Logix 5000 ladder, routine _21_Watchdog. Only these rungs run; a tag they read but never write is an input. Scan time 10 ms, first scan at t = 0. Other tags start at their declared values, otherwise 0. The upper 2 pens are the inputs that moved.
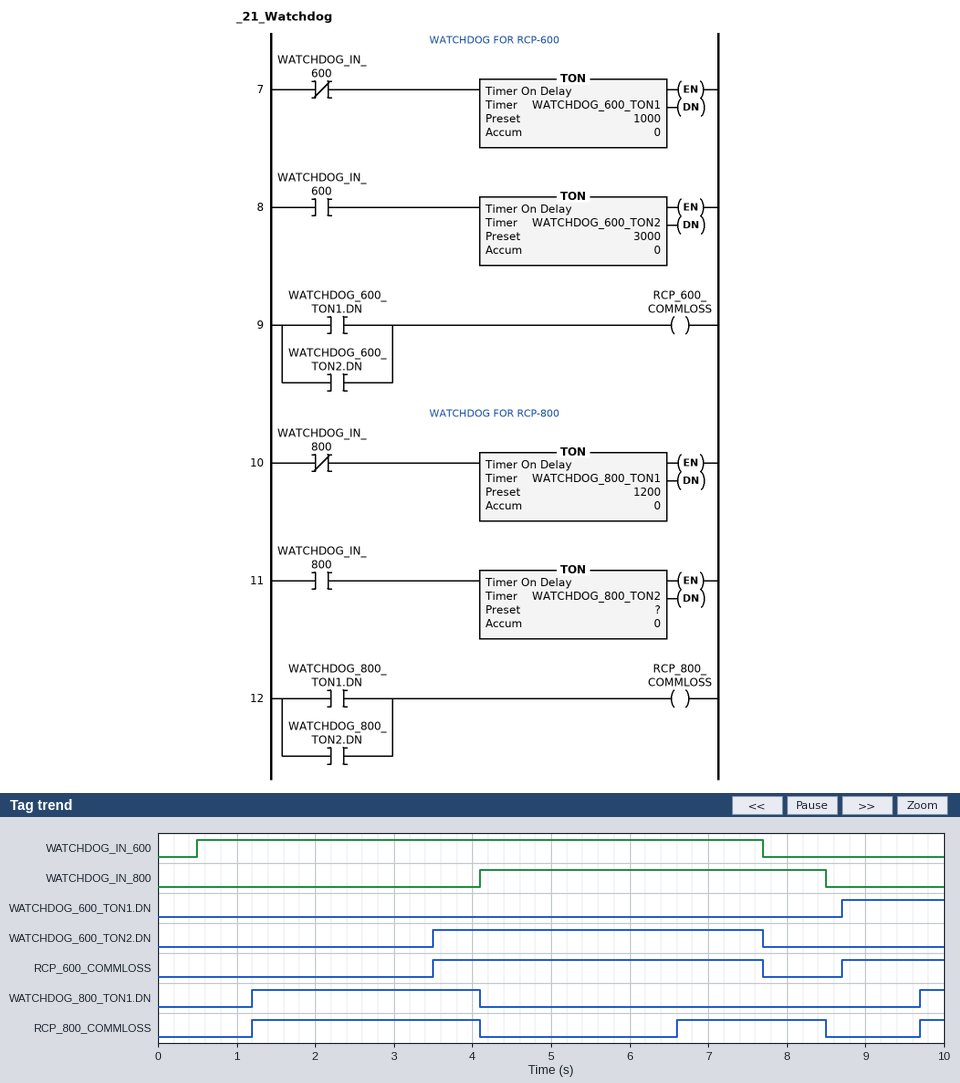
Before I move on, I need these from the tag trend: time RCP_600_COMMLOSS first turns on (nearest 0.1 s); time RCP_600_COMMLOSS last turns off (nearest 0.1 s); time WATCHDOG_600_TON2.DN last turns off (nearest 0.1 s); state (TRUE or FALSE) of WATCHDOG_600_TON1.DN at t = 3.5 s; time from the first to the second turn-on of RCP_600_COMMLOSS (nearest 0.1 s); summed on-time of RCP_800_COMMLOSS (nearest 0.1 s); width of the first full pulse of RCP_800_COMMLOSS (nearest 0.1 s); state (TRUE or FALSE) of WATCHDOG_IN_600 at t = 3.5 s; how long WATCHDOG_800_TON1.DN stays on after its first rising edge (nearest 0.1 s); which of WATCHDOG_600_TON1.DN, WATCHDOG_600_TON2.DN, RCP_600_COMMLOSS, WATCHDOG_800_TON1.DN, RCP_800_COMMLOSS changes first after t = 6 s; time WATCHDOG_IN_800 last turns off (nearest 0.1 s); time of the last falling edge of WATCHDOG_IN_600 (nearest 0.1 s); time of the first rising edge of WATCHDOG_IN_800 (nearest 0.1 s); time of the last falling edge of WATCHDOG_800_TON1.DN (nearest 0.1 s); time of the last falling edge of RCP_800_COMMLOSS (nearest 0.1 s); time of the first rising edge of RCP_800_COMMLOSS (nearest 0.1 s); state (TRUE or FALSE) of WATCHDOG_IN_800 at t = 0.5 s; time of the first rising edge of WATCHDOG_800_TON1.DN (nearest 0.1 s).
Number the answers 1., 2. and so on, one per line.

1. 3.5 s
2. 7.7 s
3. 7.7 s
4. FALSE
5. 5.2 s
6. 5.1 s
7. 2.9 s
8. TRUE
9. 2.9 s
10. RCP_800_COMMLOSS
11. 8.5 s
12. 7.7 s
13. 4.1 s
14. 4.1 s
15. 8.5 s
16. 1.2 s
17. FALSE
18. 1.2 s
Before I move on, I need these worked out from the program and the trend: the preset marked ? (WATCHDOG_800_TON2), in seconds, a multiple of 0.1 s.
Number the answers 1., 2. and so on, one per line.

1. 2.5 s
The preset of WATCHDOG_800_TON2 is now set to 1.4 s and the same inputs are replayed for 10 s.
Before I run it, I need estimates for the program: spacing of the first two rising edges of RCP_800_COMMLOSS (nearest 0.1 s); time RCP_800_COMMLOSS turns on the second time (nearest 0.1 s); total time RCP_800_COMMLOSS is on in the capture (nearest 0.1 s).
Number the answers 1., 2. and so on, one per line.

1. 4.3 s
2. 5.5 s
3. 6.2 s
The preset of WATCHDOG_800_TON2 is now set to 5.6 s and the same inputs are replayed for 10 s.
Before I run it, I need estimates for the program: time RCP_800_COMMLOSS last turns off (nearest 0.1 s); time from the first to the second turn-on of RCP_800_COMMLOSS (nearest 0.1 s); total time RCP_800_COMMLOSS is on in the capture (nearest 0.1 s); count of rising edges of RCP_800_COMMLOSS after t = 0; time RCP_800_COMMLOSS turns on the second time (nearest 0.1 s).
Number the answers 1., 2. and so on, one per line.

1. 4.1 s
2. 8.5 s
3. 3.2 s
4. 2
5. 9.7 s
